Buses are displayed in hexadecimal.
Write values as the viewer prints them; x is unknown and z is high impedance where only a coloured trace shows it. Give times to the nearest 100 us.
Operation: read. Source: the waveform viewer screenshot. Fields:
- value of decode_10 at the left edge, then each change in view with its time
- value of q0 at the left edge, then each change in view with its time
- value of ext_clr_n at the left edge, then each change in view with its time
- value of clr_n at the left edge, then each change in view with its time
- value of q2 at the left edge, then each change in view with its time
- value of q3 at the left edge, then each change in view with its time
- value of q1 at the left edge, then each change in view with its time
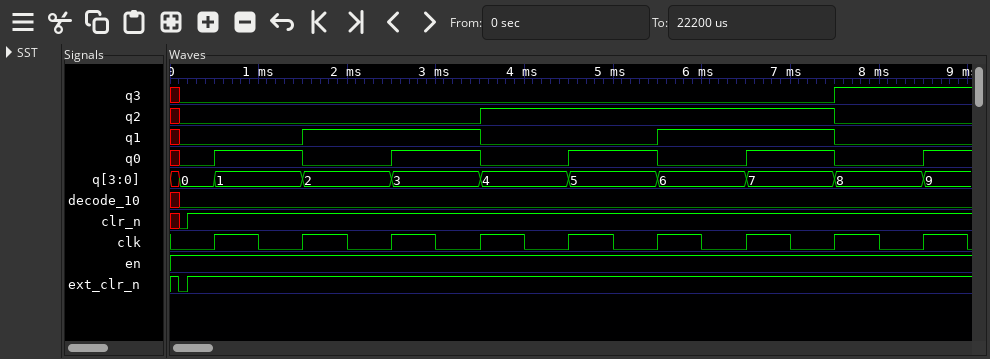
x, 0 at 100 us
x, 0 at 100 us, 1 at 500 us, 0 at 1500 us, 1 at 2500 us, 0 at 3500 us, 1 at 4500 us, 0 at 5500 us, 1 at 6500 us, 0 at 7500 us, 1 at 8500 us
1, 0 at 100 us, 1 at 200 us
x, 0 at 100 us, 1 at 200 us
x, 0 at 100 us, 1 at 3500 us, 0 at 7500 us
x, 0 at 100 us, 1 at 7500 us
x, 0 at 100 us, 1 at 1500 us, 0 at 3500 us, 1 at 5500 us, 0 at 7500 us
